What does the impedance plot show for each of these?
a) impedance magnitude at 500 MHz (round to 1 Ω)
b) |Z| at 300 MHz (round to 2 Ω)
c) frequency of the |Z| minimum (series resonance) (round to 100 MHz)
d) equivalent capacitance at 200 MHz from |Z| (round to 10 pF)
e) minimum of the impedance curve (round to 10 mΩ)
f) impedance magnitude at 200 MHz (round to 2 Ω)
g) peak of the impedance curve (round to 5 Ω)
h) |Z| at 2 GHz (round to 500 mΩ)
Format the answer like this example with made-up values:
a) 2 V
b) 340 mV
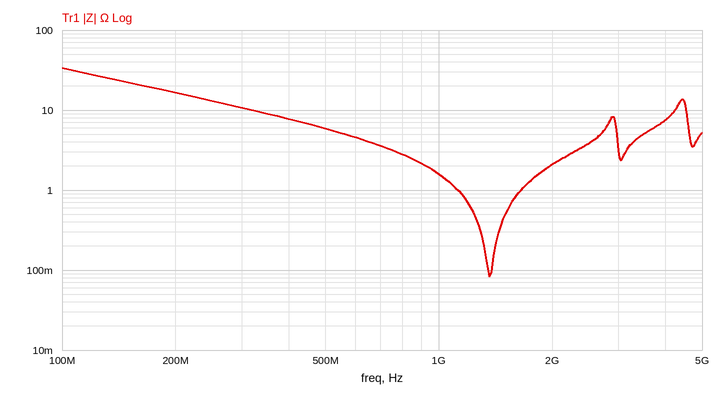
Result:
a) 6 Ω
b) 10 Ω
c) 1.4 GHz
d) 50 pF
e) 80 mΩ
f) 16 Ω
g) 35 Ω
h) 2.0 Ω
